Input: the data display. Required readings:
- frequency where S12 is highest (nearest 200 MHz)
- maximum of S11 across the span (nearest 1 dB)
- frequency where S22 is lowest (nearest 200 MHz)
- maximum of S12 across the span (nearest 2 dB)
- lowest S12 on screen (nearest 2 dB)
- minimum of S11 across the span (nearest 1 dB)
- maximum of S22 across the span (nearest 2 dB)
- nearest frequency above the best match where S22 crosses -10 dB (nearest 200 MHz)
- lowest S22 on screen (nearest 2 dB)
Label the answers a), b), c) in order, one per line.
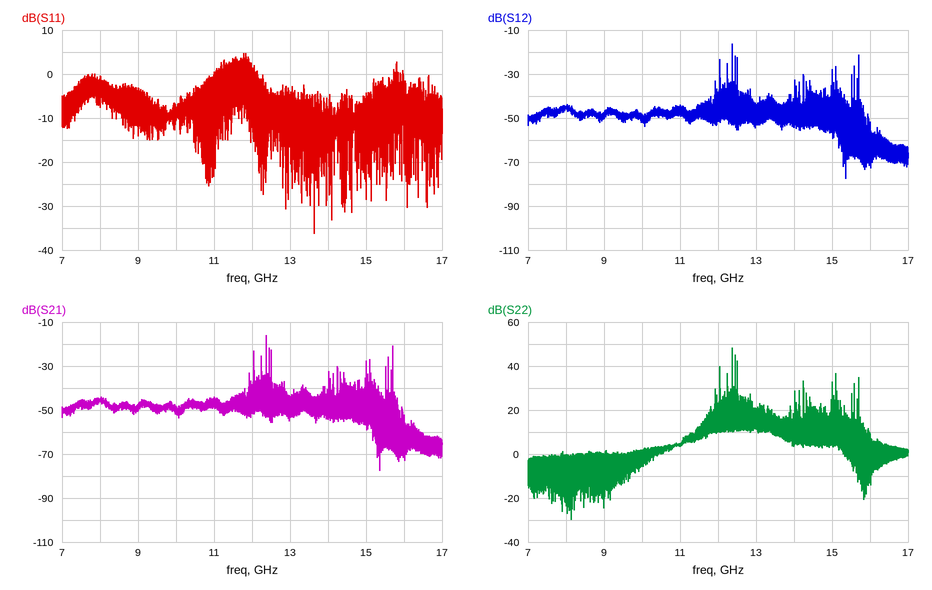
a) 12.4 GHz
b) 5 dB
c) 8.2 GHz
d) -16 dB
e) -78 dB
f) -36 dB
g) 48 dB
h) 8.2 GHz
i) -30 dB
